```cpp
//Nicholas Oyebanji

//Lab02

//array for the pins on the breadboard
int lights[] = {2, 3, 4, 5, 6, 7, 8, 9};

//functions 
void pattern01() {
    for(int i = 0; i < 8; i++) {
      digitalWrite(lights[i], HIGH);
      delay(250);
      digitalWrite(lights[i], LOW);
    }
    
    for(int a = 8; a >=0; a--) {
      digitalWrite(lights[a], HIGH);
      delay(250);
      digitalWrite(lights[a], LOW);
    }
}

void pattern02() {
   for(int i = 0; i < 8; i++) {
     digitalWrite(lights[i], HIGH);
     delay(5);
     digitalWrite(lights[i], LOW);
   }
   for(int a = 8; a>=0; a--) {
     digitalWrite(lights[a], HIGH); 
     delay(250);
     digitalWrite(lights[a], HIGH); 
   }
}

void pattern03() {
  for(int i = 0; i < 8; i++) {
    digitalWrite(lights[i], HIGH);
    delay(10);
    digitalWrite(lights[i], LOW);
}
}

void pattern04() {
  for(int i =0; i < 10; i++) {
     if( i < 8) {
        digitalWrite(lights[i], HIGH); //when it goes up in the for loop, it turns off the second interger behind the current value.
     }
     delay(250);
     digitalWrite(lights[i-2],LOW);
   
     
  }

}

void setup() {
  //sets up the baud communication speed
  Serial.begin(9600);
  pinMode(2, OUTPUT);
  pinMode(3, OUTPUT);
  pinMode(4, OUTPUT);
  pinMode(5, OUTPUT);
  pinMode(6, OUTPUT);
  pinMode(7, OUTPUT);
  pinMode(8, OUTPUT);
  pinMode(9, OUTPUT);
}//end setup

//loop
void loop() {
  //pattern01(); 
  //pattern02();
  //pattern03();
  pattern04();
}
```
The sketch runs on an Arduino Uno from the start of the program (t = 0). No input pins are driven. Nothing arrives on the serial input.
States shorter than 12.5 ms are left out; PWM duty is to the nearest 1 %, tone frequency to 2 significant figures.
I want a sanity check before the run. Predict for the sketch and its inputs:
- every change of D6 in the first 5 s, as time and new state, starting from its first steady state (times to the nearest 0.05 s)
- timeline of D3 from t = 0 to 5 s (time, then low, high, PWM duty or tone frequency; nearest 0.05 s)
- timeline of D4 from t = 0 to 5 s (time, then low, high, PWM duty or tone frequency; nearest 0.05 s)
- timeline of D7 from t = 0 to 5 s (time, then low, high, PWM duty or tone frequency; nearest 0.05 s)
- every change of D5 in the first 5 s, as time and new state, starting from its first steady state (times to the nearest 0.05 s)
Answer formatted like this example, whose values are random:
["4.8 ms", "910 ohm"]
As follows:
["0 s low; 1 s high; 1.75 s low; 3.5 s high; 4.25 s low", "0 s low; 0.25 s high; 1 s low; 2.75 s high; 3.5 s low", "0 s low; 0.5 s high; 1.25 s low; 3 s high; 3.75 s low", "0 s low; 1.25 s high; 2 s low; 3.75 s high; 4.5 s low", "0 s low; 0.75 s high; 1.5 s low; 3.25 s high; 4 s low"]
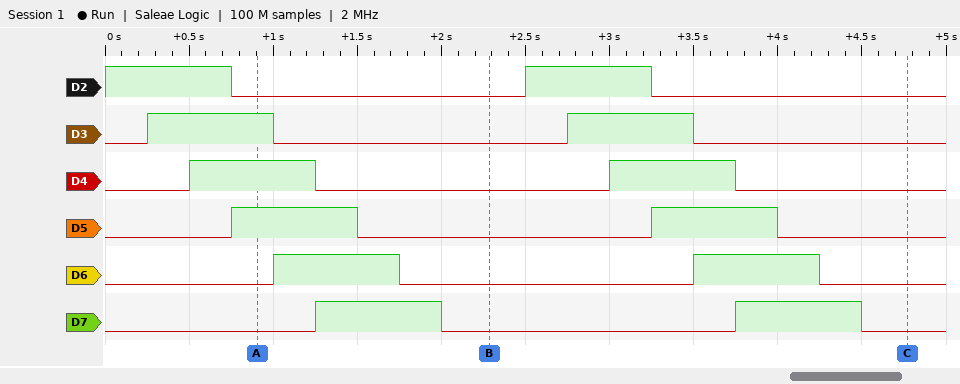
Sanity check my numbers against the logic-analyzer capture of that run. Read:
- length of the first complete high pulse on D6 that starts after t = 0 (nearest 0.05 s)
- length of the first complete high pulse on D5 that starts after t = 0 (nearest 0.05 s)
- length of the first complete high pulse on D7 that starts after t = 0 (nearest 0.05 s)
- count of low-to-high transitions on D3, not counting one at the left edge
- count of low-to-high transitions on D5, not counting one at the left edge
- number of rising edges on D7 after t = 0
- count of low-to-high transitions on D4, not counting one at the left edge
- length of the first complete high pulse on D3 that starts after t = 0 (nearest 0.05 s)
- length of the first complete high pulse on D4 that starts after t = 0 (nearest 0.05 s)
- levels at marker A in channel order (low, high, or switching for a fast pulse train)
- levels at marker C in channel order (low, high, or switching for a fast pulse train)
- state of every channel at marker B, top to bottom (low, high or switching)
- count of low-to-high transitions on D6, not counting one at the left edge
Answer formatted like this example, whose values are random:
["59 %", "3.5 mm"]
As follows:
["0.75 s", "0.75 s", "0.75 s", "2", "2", "2", "2", "0.75 s", "0.75 s", "D2 low, D3 high, D4 high, D5 high, D6 low, D7 low", "D2 low, D3 low, D4 low, D5 low, D6 low, D7 low", "D2 low, D3 low, D4 low, D5 low, D6 low, D7 low", "2"]
